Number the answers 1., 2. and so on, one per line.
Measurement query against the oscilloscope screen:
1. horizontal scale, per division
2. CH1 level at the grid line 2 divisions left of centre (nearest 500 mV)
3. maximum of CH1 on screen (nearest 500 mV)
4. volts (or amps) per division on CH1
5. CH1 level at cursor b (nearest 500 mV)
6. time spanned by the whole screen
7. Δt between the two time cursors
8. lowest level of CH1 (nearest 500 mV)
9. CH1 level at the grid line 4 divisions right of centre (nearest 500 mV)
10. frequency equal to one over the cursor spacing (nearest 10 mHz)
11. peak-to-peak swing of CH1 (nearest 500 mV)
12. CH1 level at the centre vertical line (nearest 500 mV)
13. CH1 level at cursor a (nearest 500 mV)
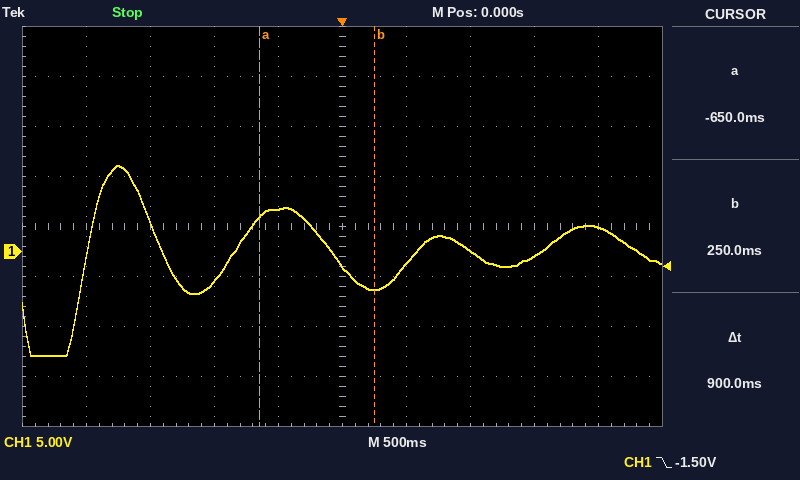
1. 500 ms
2. -3.0 V
3. 8.5 V
4. 5 V
5. -4.0 V
6. 5 s
7. 900 ms
8. -10.5 V
9. 2.5 V
10. 1.11 Hz
11. 19.0 V
12. -1.5 V
13. 3.5 V
